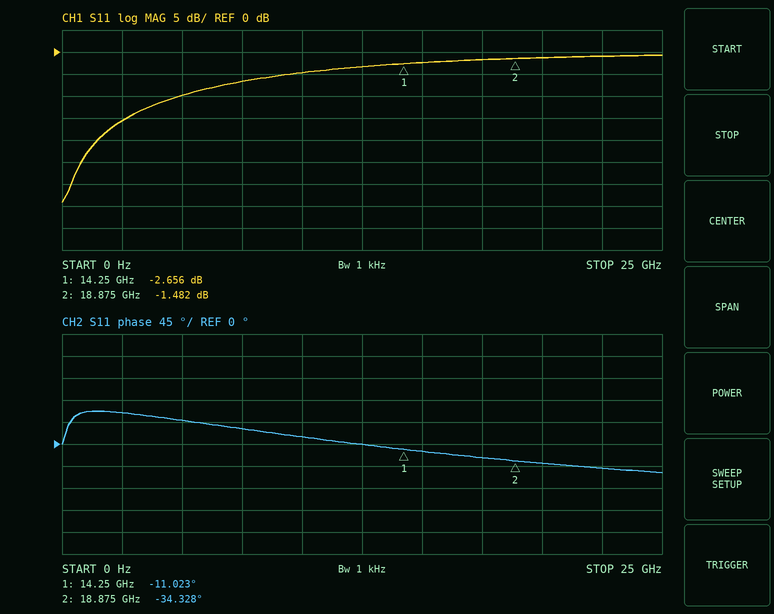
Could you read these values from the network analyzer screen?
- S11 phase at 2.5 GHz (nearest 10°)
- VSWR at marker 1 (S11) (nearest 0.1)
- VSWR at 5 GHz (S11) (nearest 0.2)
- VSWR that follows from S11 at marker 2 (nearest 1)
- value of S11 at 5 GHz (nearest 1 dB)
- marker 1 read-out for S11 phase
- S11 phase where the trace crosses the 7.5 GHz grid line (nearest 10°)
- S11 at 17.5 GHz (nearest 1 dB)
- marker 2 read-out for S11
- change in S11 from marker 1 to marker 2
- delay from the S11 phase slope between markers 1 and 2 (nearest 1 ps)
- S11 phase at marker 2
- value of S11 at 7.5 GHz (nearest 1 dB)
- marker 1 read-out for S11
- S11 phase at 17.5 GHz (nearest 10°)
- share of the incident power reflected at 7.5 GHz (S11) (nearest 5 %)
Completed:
60°
6.6
2.0
12
-10 dB
-11.023°
30°
-2 dB
-1.482 dB
1.174 dB
14 ps
-34.328°
-7 dB
-2.656 dB
-30°
20 %
